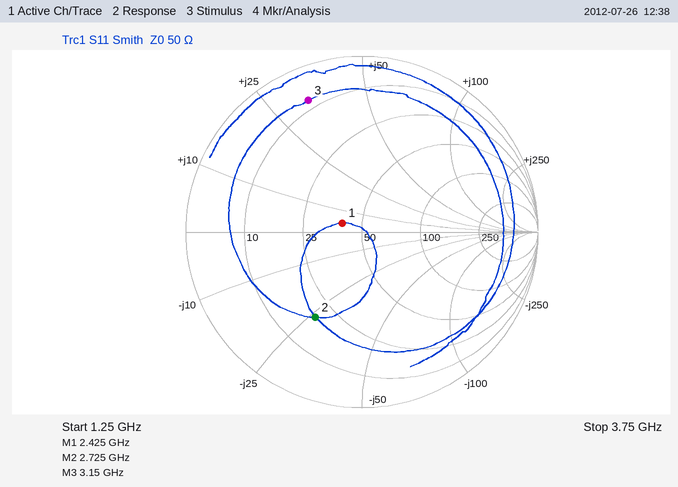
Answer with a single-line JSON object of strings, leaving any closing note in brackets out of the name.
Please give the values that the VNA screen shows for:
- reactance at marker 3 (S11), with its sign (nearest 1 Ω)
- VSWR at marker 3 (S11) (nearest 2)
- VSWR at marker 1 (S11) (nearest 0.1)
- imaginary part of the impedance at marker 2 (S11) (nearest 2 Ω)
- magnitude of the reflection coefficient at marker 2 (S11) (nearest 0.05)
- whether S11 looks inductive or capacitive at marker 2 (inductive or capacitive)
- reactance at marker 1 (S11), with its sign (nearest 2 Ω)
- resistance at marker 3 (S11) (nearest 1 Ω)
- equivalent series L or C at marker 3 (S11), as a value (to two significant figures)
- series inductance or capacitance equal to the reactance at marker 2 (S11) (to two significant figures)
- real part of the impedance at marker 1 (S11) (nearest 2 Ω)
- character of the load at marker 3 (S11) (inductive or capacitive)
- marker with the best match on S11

{"reactance at marker 3 (S11), with its sign": "+33 Ω", "VSWR at marker 3 (S11)": "10", "VSWR at marker 1 (S11)": "1.3", "imaginary part of the impedance at marker 2 (S11)": "-26 Ω", "magnitude of the reflection coefficient at marker 2 (S11)": "0.55", "whether S11 looks inductive or capacitive at marker 2": "capacitive", "reactance at marker 1 (S11), with its sign": "+4 Ω", "resistance at marker 3 (S11)": "8 Ω", "equivalent series L or C at marker 3 (S11), as a value": "1.7 nH", "series inductance or capacitance equal to the reactance at marker 2 (S11)": "2.2 pF", "real part of the impedance at marker 1 (S11)": "40 Ω", "character of the load at marker 3 (S11)": "inductive", "marker with the best match on S11": "marker 1"}
